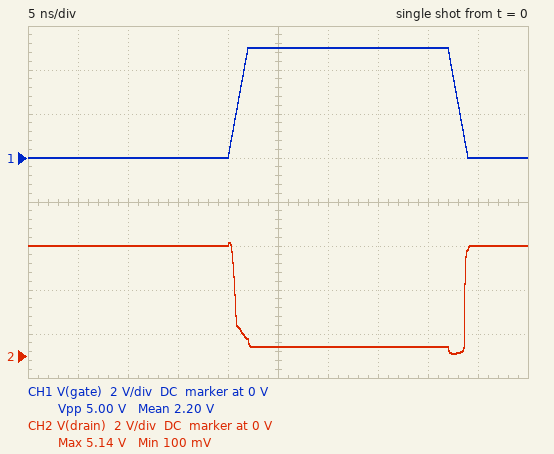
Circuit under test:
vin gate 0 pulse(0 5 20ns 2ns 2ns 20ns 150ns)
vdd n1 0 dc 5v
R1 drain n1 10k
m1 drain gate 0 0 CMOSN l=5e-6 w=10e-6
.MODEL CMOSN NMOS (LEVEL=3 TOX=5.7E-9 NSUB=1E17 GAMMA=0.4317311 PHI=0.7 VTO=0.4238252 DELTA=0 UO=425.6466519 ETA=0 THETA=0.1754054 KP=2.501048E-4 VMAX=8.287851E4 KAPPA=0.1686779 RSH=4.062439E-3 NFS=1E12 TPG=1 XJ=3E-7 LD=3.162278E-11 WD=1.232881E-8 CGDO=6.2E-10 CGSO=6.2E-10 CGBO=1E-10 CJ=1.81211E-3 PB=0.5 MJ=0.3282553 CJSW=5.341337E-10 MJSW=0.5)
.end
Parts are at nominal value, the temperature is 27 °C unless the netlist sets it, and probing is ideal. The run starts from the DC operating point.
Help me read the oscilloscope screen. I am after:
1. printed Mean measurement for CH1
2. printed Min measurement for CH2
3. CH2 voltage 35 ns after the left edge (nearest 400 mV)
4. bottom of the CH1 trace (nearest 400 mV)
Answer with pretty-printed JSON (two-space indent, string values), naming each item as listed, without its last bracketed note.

{
  "printed Mean measurement for CH1": "2.20 V",
  "printed Min measurement for CH2": "100 mV",
  "CH2 voltage 35 ns after the left edge": "400 mV",
  "bottom of the CH1 trace": "0 V"
}
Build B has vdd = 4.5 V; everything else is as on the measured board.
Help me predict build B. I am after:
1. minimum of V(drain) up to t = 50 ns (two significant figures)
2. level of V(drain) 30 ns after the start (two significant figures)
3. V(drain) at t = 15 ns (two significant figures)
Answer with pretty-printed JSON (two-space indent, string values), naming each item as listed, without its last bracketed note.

{
  "minimum of V(drain) up to t = 50 ns": "55 mV",
  "level of V(drain) 30 ns after the start": "350 mV",
  "V(drain) at t = 15 ns": "4.5 V"
}
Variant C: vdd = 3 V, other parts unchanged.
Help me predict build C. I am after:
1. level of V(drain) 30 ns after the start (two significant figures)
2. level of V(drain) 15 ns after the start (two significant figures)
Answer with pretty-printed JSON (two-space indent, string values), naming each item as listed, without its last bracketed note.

{
  "level of V(drain) 30 ns after the start": "230 mV",
  "level of V(drain) 15 ns after the start": "3.0 V"
}
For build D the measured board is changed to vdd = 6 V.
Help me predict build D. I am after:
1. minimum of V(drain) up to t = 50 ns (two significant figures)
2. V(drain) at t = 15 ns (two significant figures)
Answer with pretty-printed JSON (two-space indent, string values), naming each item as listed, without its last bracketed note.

{
  "minimum of V(drain) up to t = 50 ns": "190 mV",
  "V(drain) at t = 15 ns": "6.0 V"
}
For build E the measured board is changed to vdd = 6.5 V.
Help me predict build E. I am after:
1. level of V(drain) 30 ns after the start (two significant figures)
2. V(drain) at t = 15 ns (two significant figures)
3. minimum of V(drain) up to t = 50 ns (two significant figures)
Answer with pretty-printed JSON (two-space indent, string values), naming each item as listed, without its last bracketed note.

{
  "level of V(drain) 30 ns after the start": "520 mV",
  "V(drain) at t = 15 ns": "6.5 V",
  "minimum of V(drain) up to t = 50 ns": "240 mV"
}
